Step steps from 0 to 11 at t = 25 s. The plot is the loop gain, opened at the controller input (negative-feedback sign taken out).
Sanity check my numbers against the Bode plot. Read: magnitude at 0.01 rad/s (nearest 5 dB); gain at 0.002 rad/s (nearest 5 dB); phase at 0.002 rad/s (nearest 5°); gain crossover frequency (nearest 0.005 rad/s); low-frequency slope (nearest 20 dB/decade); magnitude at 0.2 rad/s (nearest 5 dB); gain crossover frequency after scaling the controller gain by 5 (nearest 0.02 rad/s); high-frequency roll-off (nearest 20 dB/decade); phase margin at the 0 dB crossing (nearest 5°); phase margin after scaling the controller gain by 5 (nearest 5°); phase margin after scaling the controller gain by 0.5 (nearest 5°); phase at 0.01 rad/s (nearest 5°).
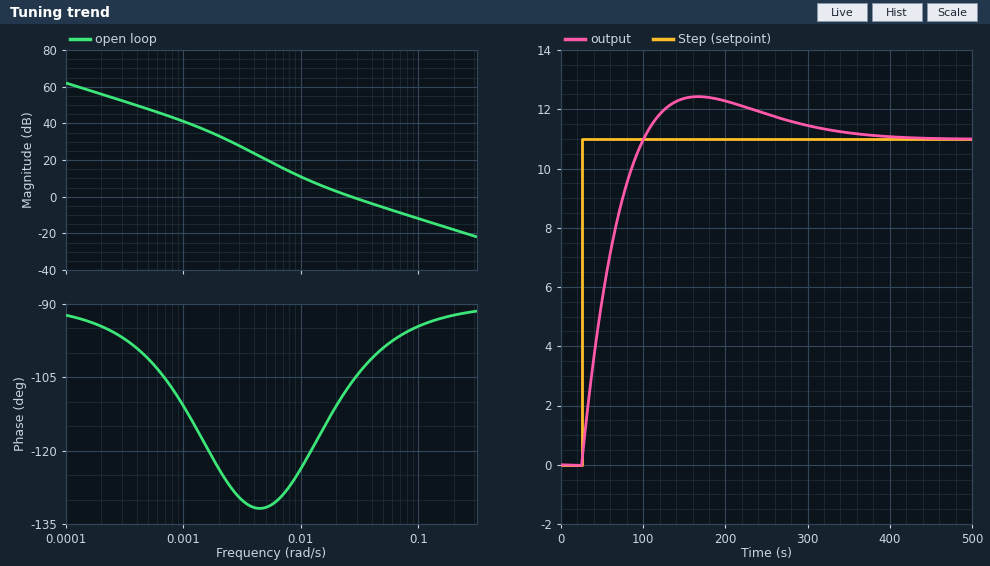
10 dB
35 dB
-125°
0.025 rad/s
-20 dB/decade
-20 dB
0.12 rad/s
-20 dB/decade
75°
85°
65°
-125°
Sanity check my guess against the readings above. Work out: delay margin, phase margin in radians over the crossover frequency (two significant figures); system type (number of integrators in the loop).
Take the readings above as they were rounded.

52 s
1
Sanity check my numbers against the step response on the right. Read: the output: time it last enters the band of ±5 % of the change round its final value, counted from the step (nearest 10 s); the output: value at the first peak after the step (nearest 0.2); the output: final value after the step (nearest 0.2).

260 s
12.4
11.0
